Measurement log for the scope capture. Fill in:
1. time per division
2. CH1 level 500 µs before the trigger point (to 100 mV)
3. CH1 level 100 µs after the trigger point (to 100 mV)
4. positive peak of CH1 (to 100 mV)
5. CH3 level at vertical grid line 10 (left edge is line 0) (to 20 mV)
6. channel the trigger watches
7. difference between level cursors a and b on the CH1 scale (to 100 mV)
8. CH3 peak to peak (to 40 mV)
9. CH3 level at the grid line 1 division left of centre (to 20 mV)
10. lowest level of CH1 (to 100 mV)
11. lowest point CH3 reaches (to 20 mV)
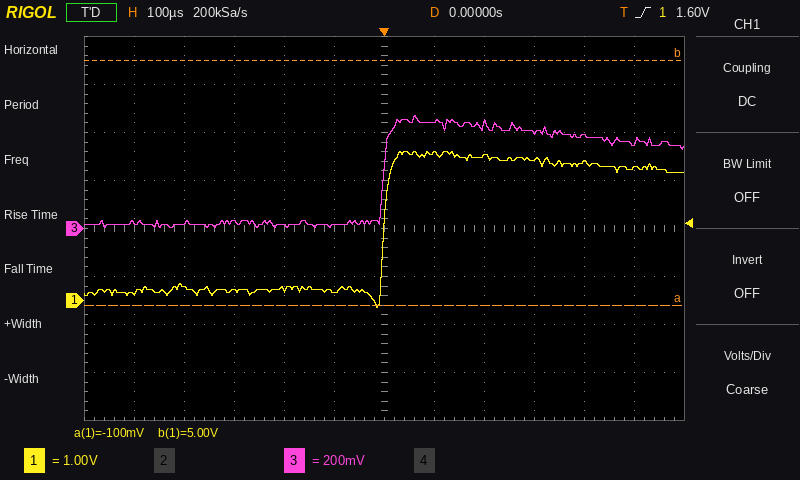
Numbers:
100 µs
200 mV
3.1 V
3.1 V
380 mV
CH1
5.1 V
480 mV
20 mV
-100 mV
0 mV
